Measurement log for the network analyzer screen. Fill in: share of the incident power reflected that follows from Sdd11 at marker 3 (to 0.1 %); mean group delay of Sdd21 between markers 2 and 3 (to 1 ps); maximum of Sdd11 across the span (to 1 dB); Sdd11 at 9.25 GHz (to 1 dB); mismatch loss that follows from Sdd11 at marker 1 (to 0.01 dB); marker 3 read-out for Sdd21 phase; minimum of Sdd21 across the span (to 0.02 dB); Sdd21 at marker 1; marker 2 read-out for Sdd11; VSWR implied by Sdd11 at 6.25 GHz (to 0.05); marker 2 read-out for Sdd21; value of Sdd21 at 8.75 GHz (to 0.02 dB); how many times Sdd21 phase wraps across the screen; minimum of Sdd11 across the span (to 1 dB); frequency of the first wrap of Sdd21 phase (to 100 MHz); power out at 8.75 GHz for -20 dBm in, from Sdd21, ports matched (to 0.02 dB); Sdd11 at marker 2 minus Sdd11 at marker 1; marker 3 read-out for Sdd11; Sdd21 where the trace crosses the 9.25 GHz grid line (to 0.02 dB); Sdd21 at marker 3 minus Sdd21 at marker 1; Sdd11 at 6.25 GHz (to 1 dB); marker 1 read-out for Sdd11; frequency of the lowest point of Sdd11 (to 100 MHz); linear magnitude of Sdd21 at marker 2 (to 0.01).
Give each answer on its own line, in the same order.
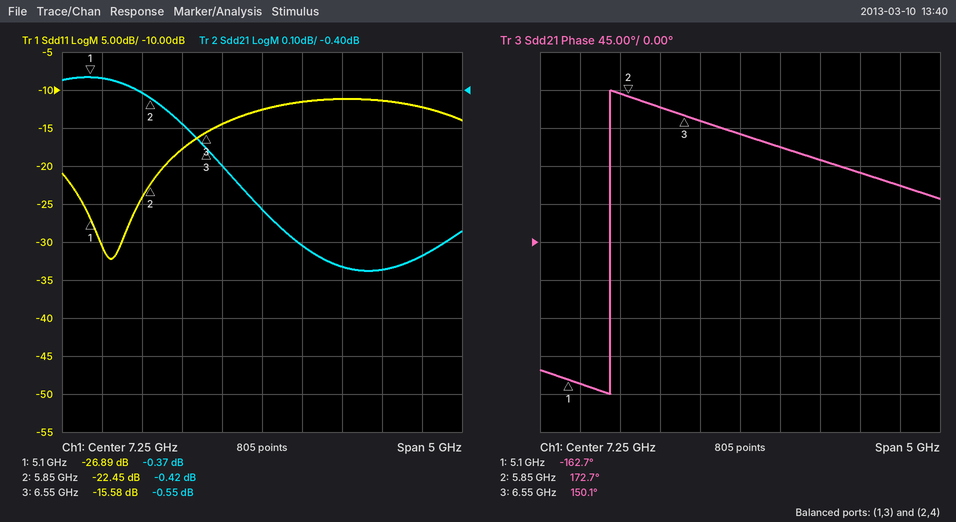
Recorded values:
2.8 %
90 ps
-11 dB
-12 dB
0.01 dB
150.1°
-0.88 dB
-0.37 dB
-22.45 dB
1.30
-0.42 dB
-0.88 dB
1
-32 dB
5.6 GHz
-20.88 dBm
4.44 dB
-15.58 dB
-0.84 dB
-0.18 dB
-18 dB
-26.89 dB
5.4 GHz
0.95
